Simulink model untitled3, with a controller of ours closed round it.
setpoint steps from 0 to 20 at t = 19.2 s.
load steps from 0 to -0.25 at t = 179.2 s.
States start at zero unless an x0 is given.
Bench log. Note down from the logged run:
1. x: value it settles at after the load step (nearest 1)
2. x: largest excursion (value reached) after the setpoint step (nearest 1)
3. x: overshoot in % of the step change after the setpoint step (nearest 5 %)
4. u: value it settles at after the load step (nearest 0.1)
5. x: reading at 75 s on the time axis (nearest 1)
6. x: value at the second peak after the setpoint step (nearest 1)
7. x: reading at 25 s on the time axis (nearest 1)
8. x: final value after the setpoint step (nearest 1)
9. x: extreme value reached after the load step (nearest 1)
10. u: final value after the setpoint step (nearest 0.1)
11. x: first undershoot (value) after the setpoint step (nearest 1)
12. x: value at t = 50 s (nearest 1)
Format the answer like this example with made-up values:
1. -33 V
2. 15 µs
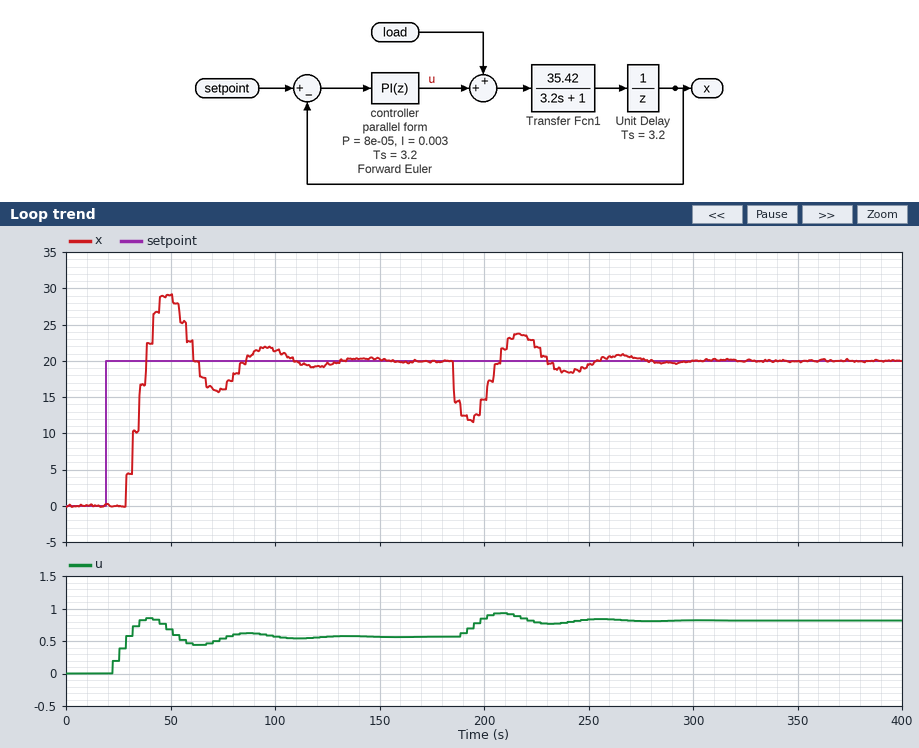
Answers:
1. 20
2. 29
3. 45 %
4. 0.8
5. 16
6. 22
7. 0
8. 20
9. 12
10. 0.6
11. 16
12. 29
